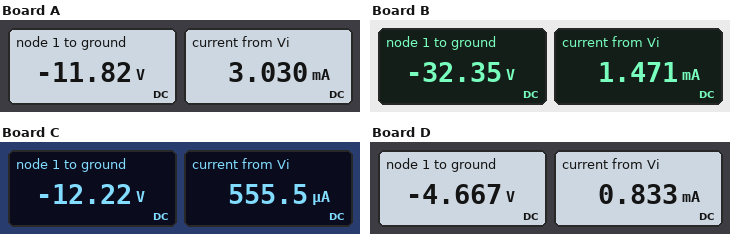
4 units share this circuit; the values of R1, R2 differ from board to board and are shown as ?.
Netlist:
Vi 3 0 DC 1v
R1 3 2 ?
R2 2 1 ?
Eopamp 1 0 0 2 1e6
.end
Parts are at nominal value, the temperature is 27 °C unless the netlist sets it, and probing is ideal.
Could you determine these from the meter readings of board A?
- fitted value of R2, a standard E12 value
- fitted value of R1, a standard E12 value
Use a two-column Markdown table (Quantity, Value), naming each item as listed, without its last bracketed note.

| Quantity | Value |
|---|---|
| fitted value of R2, a standard E12 value | 3.9 kΩ |
| fitted value of R1, a standard E12 value | 330 Ω |
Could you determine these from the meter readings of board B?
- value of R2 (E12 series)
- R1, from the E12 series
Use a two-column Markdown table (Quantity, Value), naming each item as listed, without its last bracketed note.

| Quantity | Value |
|---|---|
| value of R2 | 22 kΩ |
| R1, from the E12 series | 680 Ω |
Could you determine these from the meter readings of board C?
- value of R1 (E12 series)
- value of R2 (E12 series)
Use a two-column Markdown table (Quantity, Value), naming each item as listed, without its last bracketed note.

| Quantity | Value |
|---|---|
| value of R1 | 1.8 kΩ |
| value of R2 | 22 kΩ |
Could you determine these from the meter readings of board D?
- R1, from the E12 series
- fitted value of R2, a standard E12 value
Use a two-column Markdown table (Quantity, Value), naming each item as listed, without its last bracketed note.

| Quantity | Value |
|---|---|
| R1, from the E12 series | 1.2 kΩ |
| fitted value of R2, a standard E12 value | 5.6 kΩ |
